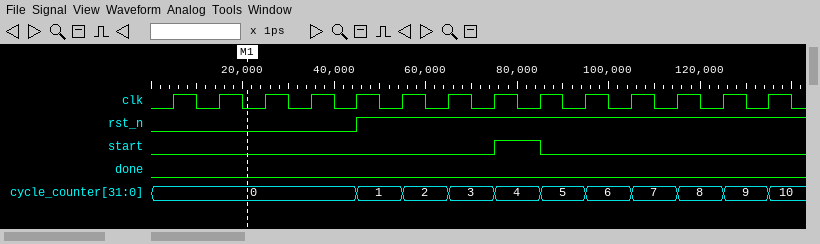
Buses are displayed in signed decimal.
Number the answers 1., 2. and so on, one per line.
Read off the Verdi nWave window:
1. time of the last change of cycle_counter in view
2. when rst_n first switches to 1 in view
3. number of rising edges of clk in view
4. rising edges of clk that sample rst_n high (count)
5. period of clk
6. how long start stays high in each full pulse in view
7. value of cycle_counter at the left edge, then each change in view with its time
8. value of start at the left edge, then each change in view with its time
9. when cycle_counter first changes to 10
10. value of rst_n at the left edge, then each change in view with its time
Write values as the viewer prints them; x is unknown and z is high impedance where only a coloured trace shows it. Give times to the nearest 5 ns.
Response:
1. 135 ns
2. 45 ns
3. 14
4. 9
5. 10 ns
6. 10 ns
7. 0, 1 at 45 ns, 2 at 55 ns, 3 at 65 ns, 4 at 75 ns, 5 at 85 ns, 6 at 95 ns, 7 at 105 ns, 8 at 115 ns, 9 at 125 ns, 10 at 135 ns
8. 0, 1 at 75 ns, 0 at 85 ns
9. 135 ns
10. 0, 1 at 45 ns
